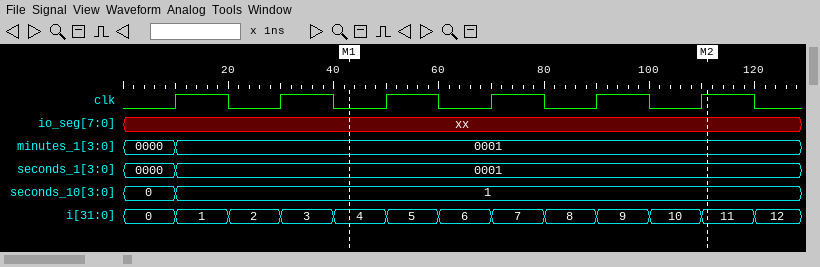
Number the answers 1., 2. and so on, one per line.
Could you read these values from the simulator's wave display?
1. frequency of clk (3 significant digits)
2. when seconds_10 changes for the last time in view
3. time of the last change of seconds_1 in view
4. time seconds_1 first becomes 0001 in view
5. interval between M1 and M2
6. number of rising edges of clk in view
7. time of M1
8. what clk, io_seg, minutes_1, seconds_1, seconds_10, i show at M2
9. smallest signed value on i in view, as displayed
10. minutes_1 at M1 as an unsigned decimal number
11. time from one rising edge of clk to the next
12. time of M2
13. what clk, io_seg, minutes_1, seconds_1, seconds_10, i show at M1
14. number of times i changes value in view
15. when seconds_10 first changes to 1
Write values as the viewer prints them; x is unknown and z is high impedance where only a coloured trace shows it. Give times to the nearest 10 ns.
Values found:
1. 50.0 MHz
2. 10 ns
3. 10 ns
4. 10 ns
5. 70 ns
6. 6
7. 40 ns
8. clk=1, io_seg=xx, minutes_1=0001, seconds_1=0001, seconds_10=1, i=11
9. 0
10. 1
11. 20 ns
12. 110 ns
13. clk=0, io_seg=xx, minutes_1=0001, seconds_1=0001, seconds_10=1, i=4
14. 12
15. 10 ns
